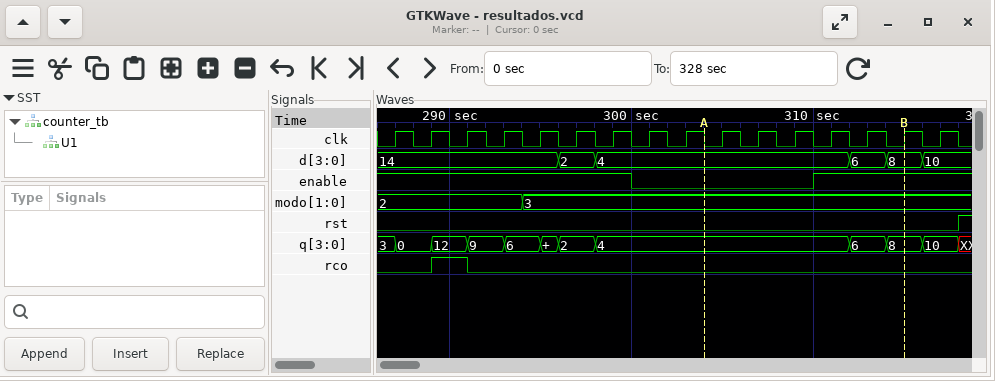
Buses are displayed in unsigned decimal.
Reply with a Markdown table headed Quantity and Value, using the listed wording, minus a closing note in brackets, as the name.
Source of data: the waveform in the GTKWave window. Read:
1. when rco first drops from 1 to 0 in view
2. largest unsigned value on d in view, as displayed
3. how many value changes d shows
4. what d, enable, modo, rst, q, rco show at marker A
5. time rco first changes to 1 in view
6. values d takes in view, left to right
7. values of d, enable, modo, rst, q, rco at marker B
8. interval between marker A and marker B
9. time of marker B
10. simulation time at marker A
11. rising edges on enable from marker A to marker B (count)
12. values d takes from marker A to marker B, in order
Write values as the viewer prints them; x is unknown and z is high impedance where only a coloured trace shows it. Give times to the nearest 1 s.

| Quantity | Value |
|---|---|
| when rco first drops from 1 to 0 in view | 291 s |
| largest unsigned value on d in view, as displayed | 14 |
| how many value changes d shows | 5 |
| what d, enable, modo, rst, q, rco show at marker A | d=4, enable=0, modo=3, rst=0, q=4, rco=0 |
| time rco first changes to 1 in view | 289 s |
| values d takes in view, left to right | 14, 2, 4, 6, 8, 10 |
| values of d, enable, modo, rst, q, rco at marker B | d=8, enable=1, modo=3, rst=0, q=8, rco=0 |
| interval between marker A and marker B | 11 s |
| time of marker B | 315 s |
| simulation time at marker A | 304 s |
| rising edges on enable from marker A to marker B | 1 |
| values d takes from marker A to marker B, in order | 4, 6, 8 |
